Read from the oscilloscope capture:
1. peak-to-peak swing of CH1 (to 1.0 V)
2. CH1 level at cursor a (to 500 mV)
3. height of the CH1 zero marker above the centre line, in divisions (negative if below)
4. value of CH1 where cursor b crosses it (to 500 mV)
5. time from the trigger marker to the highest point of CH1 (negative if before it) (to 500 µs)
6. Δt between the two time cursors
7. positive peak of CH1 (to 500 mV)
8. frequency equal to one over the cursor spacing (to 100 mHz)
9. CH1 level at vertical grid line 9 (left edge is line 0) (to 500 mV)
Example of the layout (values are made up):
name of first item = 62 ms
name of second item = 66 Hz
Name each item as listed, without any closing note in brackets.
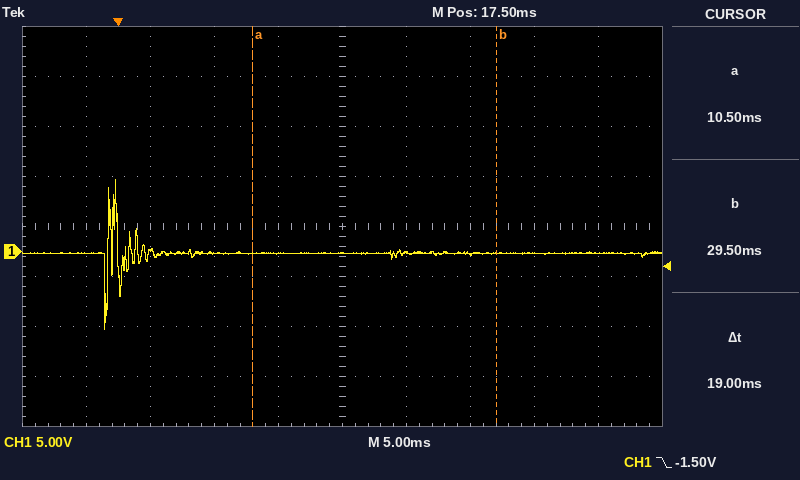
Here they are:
peak-to-peak swing of CH1 = 15.0 V
CH1 level at cursor a = 0.0 V
height of the CH1 zero marker above the centre line, in divisions = -0.5 div
value of CH1 where cursor b crosses it = 0.0 V
time from the trigger marker to the highest point of CH1 (negative if before it) = 0.0 ms
Δt between the two time cursors = 19 ms
positive peak of CH1 = 7.0 V
frequency equal to one over the cursor spacing = 52.6 Hz
CH1 level at vertical grid line 9 (left edge is line 0) = 0.0 V
